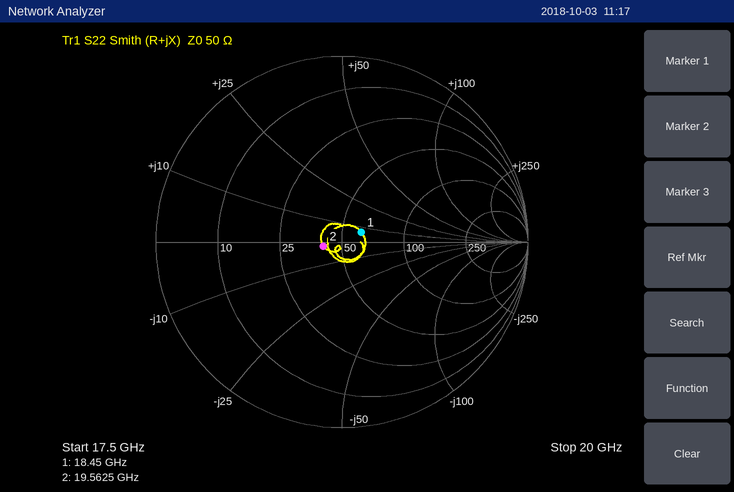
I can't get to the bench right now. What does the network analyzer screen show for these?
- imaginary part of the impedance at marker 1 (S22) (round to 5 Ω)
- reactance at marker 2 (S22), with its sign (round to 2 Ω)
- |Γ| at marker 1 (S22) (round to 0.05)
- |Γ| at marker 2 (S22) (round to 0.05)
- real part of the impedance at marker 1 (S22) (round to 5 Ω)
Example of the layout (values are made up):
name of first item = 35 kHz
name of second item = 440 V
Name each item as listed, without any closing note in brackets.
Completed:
imaginary part of the impedance at marker 1 (S22) = +5 Ω
reactance at marker 2 (S22), with its sign = -2 Ω
|Γ| at marker 1 (S22) = 0.10
|Γ| at marker 2 (S22) = 0.10
real part of the impedance at marker 1 (S22) = 60 Ω
